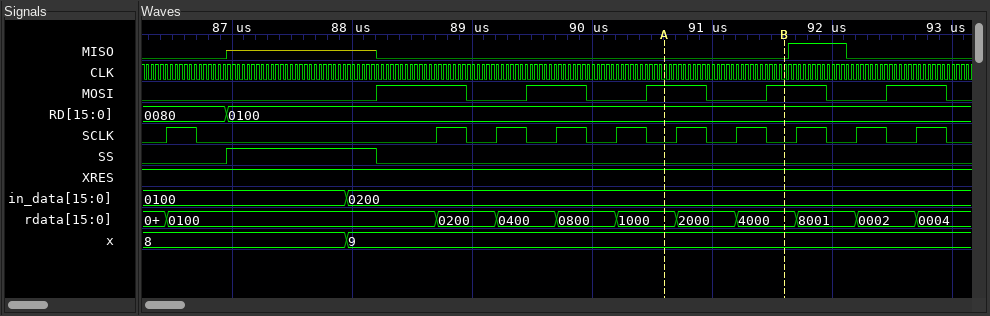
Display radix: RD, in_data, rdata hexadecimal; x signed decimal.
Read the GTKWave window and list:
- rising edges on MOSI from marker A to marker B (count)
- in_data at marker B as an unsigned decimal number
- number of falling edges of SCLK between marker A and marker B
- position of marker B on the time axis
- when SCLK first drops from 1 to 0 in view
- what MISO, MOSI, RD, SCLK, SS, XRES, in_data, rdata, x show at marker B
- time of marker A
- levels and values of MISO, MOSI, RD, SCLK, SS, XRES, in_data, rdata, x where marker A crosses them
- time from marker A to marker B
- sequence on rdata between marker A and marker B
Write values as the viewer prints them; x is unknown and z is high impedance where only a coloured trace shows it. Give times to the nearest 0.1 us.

1
512
2
91.6 us
86.7 us
MISO=0, MOSI=1, RD=0100, SCLK=0, SS=0, XRES=1, in_data=0200, rdata=4000, x=9
90.6 us
MISO=0, MOSI=1, RD=0100, SCLK=0, SS=0, XRES=1, in_data=0200, rdata=1000, x=9
1 us
1000, 2000, 4000
